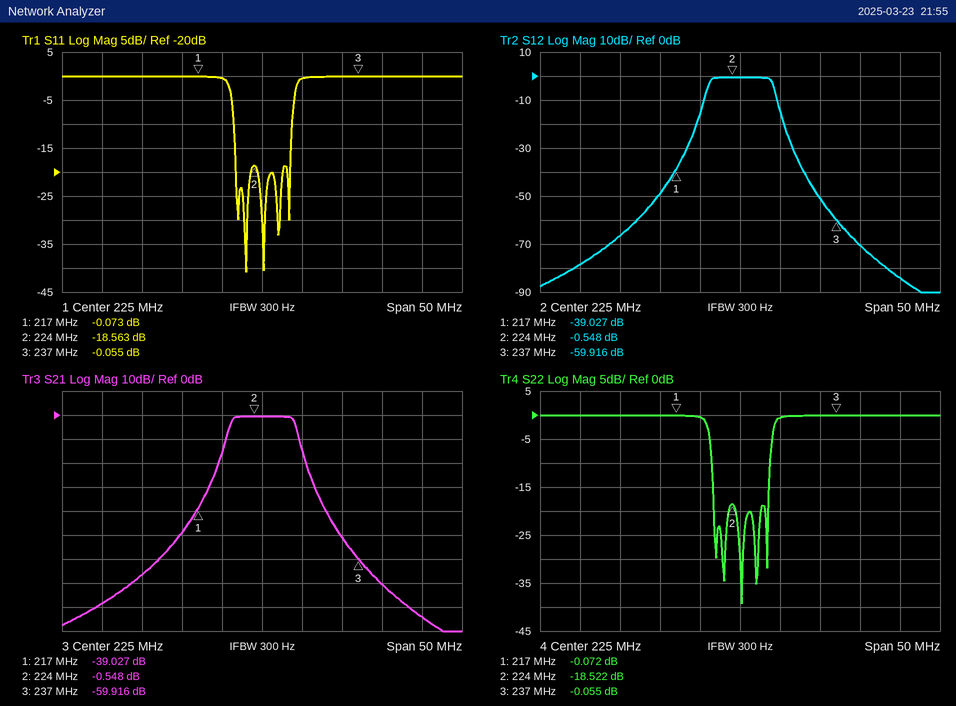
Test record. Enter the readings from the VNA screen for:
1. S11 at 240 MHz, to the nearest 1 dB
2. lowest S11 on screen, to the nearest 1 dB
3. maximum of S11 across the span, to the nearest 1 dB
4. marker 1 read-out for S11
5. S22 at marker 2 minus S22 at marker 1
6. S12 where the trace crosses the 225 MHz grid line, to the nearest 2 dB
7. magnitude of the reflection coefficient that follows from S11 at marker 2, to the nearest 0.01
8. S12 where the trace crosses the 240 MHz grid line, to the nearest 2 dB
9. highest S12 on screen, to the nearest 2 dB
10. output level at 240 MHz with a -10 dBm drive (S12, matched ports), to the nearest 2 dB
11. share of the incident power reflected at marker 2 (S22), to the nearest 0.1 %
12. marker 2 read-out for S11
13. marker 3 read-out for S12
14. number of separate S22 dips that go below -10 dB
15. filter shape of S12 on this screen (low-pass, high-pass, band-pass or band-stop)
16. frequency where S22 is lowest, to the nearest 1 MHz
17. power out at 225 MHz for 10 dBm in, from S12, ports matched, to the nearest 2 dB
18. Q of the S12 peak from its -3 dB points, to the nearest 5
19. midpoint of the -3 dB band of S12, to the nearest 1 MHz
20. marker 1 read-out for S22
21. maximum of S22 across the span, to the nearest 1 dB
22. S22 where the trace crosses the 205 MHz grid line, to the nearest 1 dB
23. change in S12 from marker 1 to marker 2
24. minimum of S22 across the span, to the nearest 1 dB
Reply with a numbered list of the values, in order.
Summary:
1. 0 dB
2. -41 dB
3. 0 dB
4. -0.073 dB
5. -18.450 dB
6. 0 dB
7. 0.12
8. -70 dB
9. 0 dB
10. -80 dBm
11. 1.4 %
12. -18.563 dB
13. -59.916 dB
14. 5
15. band-pass
16. 225 MHz
17. 10 dBm
18. 30
19. 225 MHz
20. -0.072 dB
21. 0 dB
22. 0 dB
23. 38.479 dB
24. -39 dB
